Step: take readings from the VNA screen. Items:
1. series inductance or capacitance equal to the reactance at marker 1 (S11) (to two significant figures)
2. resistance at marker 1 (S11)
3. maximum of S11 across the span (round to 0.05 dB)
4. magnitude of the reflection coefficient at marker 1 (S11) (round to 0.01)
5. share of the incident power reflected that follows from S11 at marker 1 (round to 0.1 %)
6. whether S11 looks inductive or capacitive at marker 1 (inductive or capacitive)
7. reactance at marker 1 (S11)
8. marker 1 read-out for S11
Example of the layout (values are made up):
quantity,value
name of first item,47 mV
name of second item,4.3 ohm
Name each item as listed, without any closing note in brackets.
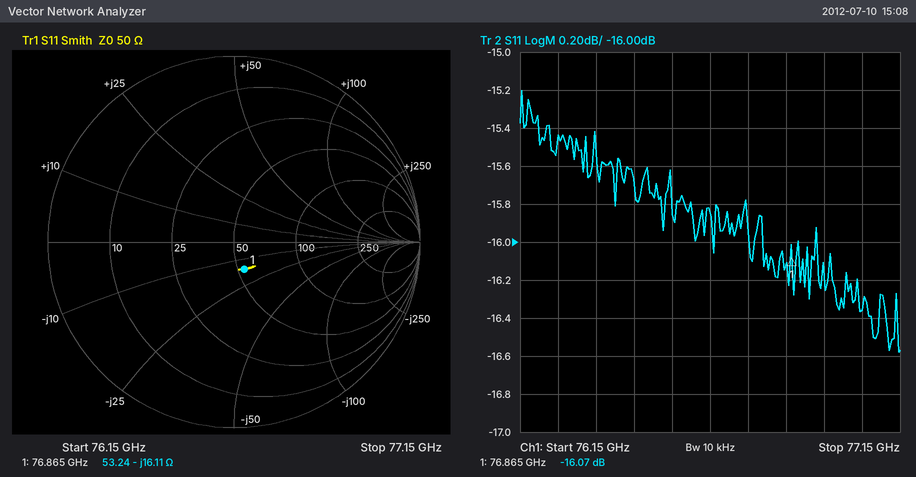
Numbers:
quantity,value
series inductance or capacitance equal to the reactance at marker 1 (S11),130 fF
resistance at marker 1,53.24 Ω
maximum of S11 across the span,-15.20 dB
magnitude of the reflection coefficient at marker 1 (S11),0.16
share of the incident power reflected that follows from S11 at marker 1,2.5 %
whether S11 looks inductive or capacitive at marker 1,capacitive
reactance at marker 1,-16.11 Ω
marker 1 read-out for S11,-16.07 dB
